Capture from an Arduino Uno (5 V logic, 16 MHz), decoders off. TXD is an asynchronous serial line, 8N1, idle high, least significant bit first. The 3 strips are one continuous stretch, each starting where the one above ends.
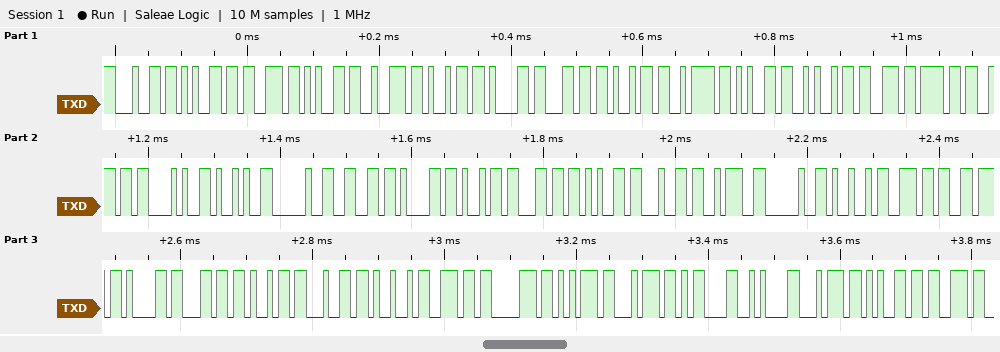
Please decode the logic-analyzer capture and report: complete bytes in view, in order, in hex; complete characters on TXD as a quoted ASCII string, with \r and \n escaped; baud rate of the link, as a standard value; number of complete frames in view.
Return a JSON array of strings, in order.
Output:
["0x64 0x65 0x73 0x65 0x72 0x69 0x61 0x6C 0x69 0x7A 0x65 0x4A 0x73 0x6F 0x6E 0x28 0x29 0x20 0x66 0x61 0x69 0x6C 0x65 0x64 0x3A 0x20 0x49 0x6E 0x76 0x61 0x6C 0x69 0x64 0x49 0x6E 0x70 0x75 0x74 0x0D 0x0A 0x74 0x65 0x73", "\"deserializeJson() failed: InvalidInput\\r\\ntes\"", "115200 baud", "43"]
